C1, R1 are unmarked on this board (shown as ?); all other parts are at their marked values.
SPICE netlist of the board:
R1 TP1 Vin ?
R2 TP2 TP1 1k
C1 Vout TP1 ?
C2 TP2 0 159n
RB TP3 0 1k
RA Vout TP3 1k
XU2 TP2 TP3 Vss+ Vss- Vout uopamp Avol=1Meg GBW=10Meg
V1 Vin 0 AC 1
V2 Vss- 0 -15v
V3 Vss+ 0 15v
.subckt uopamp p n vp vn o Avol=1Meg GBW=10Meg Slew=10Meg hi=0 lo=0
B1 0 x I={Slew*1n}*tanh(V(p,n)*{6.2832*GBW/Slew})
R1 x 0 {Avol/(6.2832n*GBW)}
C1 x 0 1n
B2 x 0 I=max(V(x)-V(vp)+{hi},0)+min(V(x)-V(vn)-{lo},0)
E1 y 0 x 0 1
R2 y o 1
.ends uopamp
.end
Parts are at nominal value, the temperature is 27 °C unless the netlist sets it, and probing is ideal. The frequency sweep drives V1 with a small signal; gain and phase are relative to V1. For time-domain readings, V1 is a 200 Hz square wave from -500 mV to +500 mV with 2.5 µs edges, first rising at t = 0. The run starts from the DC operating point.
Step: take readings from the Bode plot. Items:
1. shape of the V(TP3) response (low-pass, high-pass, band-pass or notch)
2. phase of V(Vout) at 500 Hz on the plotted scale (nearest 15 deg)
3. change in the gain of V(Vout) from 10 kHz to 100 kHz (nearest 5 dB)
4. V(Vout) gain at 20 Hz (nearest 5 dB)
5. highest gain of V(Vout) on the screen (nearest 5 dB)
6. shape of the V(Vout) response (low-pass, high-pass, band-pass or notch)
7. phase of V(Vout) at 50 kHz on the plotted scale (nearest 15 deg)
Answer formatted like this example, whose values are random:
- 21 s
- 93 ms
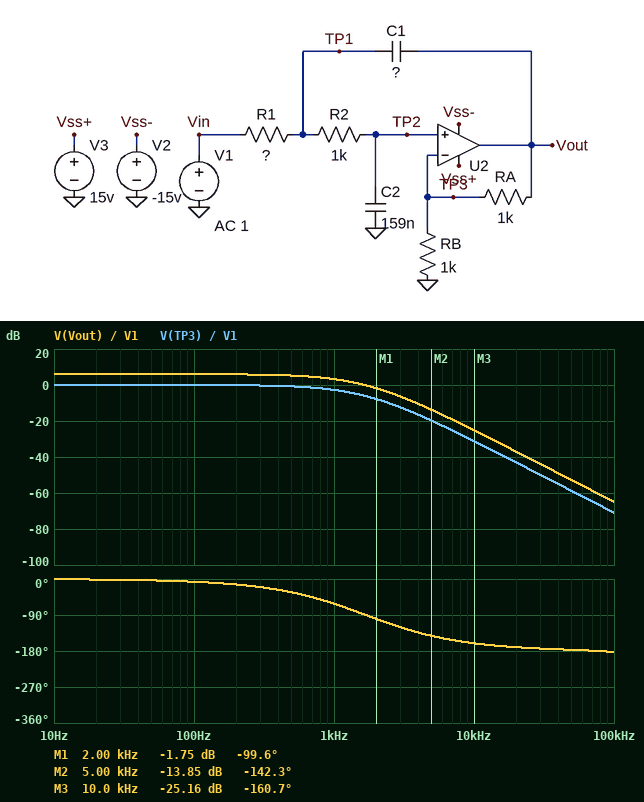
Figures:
- low-pass
- -30 deg
- -40 dB
- 5 dB
- 5 dB
- low-pass
- -180 deg
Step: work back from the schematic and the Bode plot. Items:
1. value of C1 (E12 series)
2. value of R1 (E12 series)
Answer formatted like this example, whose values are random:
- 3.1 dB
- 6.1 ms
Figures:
- 100 nF
- 560 Ω
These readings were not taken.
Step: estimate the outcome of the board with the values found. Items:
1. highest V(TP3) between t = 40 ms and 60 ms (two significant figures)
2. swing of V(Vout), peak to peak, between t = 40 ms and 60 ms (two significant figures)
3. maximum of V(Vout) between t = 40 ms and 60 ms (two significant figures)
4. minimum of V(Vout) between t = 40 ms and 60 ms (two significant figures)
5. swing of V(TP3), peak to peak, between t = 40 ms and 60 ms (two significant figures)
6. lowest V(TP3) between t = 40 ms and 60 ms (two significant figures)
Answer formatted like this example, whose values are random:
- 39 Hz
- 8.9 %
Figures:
- 500 mV
- 2.0 V
- 1.0 V
- -1.0 V
- 1.0 V
- -500 mV
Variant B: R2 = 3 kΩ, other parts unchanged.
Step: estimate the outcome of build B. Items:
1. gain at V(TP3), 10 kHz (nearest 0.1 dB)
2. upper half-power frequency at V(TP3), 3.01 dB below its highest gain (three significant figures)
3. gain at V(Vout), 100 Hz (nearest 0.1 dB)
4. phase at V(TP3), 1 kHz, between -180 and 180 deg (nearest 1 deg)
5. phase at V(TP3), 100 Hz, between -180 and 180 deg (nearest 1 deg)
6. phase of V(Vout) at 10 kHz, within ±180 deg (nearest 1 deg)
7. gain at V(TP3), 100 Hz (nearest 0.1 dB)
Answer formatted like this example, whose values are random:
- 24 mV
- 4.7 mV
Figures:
- -40.8 dB
- 347 Hz
- 5.7 dB
- -91 deg
- -18 deg
- -163 deg
- -0.3 dB
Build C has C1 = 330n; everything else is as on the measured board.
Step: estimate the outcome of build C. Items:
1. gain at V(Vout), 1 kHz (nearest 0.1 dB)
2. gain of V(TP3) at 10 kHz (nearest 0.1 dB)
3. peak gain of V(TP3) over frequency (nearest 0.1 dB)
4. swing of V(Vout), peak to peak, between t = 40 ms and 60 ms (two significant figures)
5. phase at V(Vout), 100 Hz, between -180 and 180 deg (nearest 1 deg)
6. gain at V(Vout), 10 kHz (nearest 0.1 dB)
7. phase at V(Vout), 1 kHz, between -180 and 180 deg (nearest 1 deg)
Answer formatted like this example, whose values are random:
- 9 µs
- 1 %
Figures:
- 13.4 dB
- -41.2 dB
- 8.8 dB
- 4.2 V
- -2 deg
- -35.2 dB
- -112 deg
